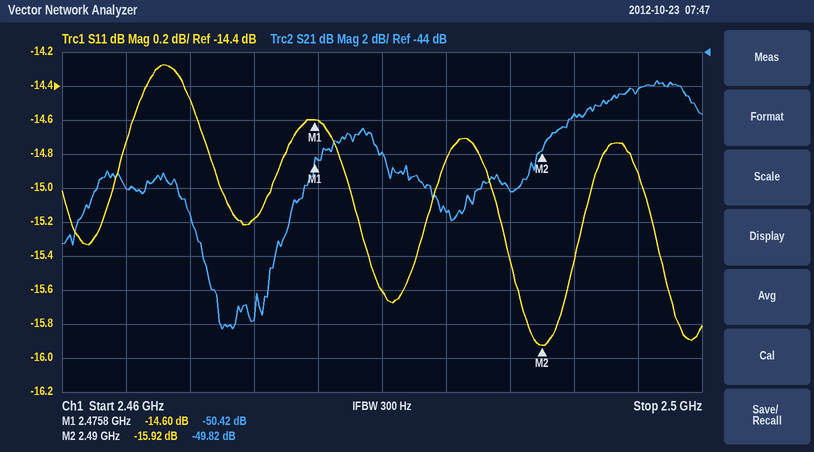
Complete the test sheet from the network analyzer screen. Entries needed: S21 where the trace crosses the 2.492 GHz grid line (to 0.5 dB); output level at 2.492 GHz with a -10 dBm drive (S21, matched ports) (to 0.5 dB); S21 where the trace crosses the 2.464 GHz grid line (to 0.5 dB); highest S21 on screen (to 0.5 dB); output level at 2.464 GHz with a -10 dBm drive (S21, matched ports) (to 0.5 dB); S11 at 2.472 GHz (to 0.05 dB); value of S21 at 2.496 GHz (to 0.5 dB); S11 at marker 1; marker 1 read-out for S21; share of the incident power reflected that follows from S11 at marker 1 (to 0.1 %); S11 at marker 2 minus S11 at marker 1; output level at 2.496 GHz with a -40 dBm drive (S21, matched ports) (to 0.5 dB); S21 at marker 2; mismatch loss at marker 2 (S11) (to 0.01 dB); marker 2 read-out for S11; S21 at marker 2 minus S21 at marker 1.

-47.5 dB
-57.5 dBm
-52.0 dB
-45.5 dB
-62.0 dBm
-15.20 dB
-46.0 dB
-14.60 dB
-50.42 dB
3.5 %
-1.32 dB
-86.0 dBm
-49.82 dB
0.11 dB
-15.92 dB
0.60 dB
